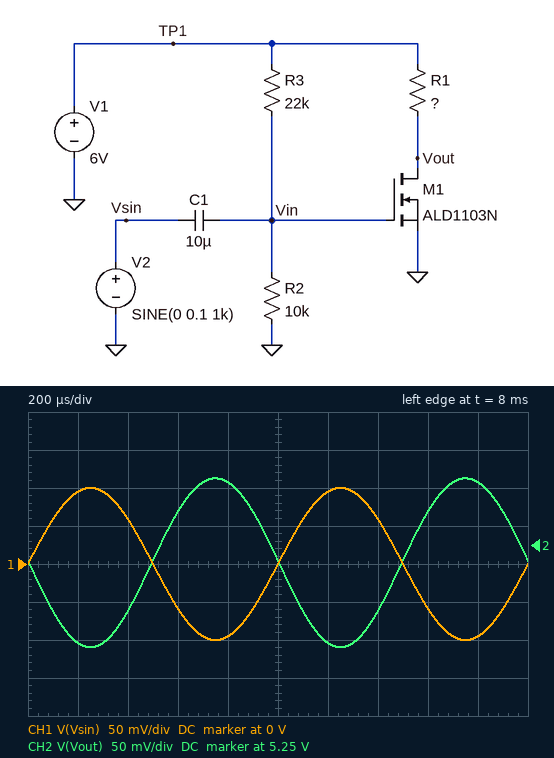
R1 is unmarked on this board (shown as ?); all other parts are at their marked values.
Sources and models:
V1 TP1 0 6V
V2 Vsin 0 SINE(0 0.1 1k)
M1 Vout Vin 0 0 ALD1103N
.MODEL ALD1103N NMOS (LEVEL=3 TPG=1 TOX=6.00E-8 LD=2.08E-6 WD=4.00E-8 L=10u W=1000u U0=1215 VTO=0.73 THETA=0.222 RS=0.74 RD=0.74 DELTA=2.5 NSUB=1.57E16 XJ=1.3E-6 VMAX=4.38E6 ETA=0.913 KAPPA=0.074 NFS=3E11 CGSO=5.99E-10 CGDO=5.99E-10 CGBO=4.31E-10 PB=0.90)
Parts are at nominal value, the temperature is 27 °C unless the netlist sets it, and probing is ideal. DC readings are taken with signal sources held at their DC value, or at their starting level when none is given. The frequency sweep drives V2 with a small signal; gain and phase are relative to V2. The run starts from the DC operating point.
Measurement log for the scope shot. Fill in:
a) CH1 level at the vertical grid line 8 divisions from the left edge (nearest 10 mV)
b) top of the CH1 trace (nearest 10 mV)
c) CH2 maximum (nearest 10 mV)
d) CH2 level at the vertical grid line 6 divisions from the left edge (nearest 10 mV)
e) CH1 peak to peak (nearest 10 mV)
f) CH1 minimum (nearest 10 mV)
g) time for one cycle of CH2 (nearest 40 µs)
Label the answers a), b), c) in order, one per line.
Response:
a) -60 mV
b) 100 mV
c) 5.34 V
d) 5.12 V
e) 200 mV
f) -100 mV
g) 1.00 ms
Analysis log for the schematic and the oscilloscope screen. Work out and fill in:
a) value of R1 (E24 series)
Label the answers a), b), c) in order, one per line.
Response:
a) 150 Ω
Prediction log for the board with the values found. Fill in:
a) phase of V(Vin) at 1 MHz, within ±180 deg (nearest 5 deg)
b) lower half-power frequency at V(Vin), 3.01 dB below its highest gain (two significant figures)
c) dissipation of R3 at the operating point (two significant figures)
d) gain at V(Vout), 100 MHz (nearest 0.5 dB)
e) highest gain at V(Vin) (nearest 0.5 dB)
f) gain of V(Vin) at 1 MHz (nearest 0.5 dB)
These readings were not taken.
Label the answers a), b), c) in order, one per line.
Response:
a) 0 deg
b) 2.3 Hz
c) 770 µW
d) 1.0 dB
e) 0 dB
f) 0 dB
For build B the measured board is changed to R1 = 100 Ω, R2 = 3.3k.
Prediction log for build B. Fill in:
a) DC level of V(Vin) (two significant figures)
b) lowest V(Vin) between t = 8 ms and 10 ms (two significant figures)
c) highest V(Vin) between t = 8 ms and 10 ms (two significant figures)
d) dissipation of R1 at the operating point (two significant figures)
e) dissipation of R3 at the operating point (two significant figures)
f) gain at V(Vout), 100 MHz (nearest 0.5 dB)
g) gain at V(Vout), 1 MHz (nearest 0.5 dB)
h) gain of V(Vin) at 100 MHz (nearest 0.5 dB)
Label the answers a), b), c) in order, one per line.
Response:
a) 780 mV
b) 680 mV
c) 880 mV
d) 630 nW
e) 1.2 mW
f) -18.5 dB
g) -19.0 dB
h) 0 dB
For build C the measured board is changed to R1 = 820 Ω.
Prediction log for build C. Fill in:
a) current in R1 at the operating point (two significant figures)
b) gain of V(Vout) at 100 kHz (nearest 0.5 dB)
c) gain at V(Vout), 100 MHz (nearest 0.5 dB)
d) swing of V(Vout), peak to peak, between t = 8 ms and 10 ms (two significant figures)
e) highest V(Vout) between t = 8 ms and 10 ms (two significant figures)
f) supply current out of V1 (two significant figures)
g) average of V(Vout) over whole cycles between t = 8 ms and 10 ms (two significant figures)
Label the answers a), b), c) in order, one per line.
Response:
a) 5.0 mA
b) 15.5 dB
c) 15.0 dB
d) 1.2 V
e) 2.5 V
f) 5.2 mA
g) 1.9 V
